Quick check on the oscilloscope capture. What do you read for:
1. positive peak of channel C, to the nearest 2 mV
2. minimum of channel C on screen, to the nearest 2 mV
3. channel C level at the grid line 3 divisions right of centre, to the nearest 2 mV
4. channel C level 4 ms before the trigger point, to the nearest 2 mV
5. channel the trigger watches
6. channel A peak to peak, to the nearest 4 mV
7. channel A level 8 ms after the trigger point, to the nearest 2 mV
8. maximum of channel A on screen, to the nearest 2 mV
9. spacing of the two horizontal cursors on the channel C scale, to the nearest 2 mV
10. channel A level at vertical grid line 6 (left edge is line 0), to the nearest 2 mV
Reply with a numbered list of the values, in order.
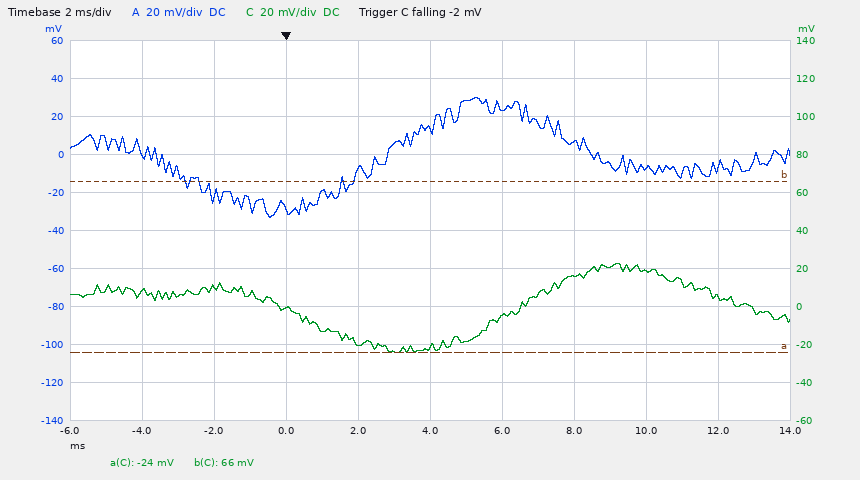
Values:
1. 22 mV
2. -24 mV
3. 18 mV
4. 8 mV
5. channel C
6. 64 mV
7. 6 mV
8. 30 mV
9. 90 mV
10. 24 mV
